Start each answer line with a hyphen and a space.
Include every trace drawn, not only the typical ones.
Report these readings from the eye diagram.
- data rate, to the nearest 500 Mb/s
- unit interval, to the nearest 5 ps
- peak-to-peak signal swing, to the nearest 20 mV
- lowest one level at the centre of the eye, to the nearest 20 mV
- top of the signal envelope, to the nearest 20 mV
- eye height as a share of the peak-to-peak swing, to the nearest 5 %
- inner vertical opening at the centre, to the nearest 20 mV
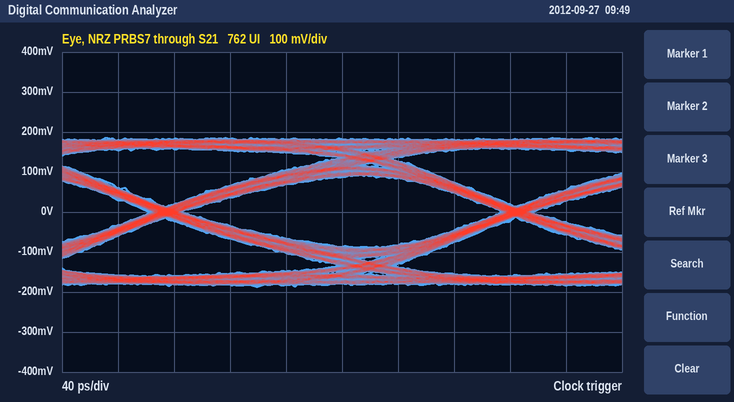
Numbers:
- 4.0 Gb/s
- 250 ps
- 380 mV
- 80 mV
- 180 mV
- 45 %
- 180 mV
